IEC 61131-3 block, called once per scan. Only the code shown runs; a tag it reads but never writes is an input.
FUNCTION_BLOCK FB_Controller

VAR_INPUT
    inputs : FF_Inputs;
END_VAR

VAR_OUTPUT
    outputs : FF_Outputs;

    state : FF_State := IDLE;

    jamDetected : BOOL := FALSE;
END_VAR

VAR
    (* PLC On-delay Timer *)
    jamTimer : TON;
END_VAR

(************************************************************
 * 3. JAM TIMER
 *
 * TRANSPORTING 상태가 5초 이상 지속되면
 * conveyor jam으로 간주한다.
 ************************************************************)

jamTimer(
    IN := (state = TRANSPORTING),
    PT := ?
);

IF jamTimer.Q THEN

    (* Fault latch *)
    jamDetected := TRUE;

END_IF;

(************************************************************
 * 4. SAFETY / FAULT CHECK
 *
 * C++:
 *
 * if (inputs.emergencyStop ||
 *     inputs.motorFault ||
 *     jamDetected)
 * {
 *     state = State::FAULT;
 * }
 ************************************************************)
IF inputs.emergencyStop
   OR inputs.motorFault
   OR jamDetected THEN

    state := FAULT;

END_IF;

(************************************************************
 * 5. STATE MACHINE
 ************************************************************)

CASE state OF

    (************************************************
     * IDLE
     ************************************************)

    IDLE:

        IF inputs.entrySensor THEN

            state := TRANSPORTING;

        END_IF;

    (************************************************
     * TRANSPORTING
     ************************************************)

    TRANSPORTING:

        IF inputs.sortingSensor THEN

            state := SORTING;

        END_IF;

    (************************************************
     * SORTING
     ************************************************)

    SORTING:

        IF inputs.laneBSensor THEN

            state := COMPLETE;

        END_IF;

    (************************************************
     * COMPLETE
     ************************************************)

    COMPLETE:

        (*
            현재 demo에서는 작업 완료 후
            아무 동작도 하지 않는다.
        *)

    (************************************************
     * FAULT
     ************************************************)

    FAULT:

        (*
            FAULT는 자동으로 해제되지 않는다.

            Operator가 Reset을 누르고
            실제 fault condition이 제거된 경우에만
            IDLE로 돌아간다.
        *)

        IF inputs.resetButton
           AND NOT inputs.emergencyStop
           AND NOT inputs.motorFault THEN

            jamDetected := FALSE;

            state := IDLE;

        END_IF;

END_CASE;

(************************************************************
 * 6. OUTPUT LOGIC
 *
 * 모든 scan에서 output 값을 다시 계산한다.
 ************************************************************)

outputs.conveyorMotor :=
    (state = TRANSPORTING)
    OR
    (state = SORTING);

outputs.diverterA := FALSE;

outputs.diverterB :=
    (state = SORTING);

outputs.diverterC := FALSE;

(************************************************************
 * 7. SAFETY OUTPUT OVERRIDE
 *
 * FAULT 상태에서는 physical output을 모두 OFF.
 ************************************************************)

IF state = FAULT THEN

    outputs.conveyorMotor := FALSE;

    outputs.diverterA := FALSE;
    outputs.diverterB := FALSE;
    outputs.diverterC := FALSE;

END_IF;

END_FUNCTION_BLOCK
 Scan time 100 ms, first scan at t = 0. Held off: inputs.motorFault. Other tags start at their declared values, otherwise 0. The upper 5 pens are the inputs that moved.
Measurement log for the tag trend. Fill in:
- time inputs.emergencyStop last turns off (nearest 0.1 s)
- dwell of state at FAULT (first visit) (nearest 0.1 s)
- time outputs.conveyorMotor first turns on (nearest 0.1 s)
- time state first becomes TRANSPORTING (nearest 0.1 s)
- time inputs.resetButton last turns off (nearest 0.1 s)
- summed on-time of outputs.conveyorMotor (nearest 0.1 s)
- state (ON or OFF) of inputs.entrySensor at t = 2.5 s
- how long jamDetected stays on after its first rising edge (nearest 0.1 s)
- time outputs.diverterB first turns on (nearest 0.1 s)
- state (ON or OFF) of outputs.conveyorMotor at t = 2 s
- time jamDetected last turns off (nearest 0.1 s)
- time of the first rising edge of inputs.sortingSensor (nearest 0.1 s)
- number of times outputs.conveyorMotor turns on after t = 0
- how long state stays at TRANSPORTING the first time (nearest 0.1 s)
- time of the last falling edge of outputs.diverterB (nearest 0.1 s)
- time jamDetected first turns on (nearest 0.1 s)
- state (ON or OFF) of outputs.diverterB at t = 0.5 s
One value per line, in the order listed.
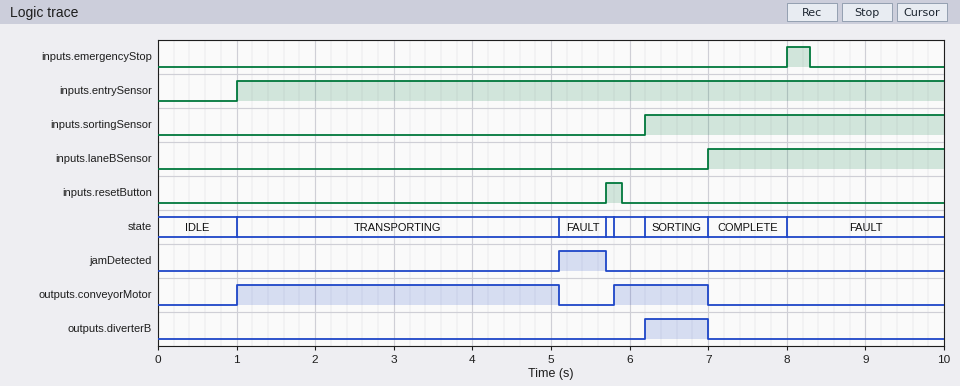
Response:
8.3 s
0.6 s
1.0 s
1.0 s
5.9 s
5.3 s
ON
0.6 s
6.2 s
ON
5.7 s
6.2 s
2
4.1 s
7.0 s
5.1 s
OFF
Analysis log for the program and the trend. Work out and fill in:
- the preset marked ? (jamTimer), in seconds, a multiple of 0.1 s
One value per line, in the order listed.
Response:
4.0 s
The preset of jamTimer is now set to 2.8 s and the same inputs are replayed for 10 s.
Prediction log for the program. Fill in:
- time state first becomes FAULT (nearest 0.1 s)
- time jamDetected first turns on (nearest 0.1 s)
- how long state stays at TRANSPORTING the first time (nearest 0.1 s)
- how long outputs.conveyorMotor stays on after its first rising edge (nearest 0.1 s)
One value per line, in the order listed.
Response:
3.9 s
3.9 s
2.9 s
2.9 s
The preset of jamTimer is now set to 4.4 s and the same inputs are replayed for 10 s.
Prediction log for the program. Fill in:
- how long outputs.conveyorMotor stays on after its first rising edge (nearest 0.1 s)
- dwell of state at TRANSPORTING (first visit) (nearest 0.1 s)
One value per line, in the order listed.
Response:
4.5 s
4.5 s
